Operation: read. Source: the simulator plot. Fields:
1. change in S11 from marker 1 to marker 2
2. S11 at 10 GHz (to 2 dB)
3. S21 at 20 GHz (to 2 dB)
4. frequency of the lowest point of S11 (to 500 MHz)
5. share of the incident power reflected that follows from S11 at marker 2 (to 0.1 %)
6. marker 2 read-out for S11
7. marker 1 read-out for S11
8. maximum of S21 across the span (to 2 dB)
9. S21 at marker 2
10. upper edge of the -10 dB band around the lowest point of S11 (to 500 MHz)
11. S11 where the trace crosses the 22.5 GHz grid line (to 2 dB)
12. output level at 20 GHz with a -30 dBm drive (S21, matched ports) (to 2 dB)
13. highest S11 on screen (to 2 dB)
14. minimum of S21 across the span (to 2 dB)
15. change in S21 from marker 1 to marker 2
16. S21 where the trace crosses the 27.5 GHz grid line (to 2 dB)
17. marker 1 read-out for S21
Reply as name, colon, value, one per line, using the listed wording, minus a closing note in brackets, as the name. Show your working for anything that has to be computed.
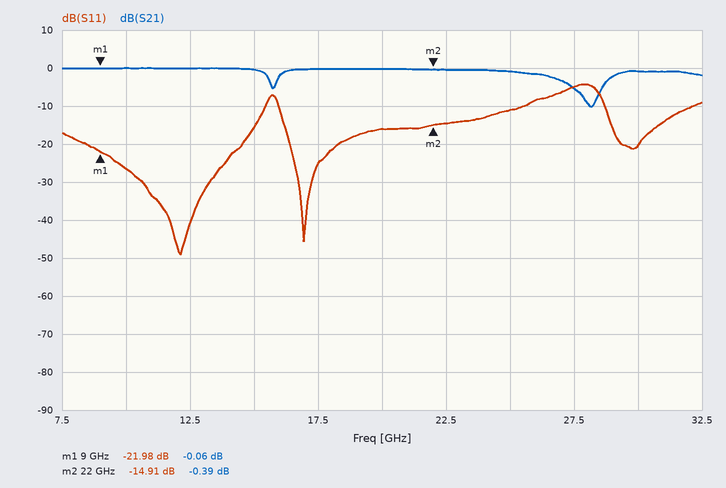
change in S11 from marker 1 to marker 2: -14.91 − (-21.98) = 7.07 dB
S11 at 10 GHz: -26 dB
S21 at 20 GHz: 0 dB
frequency of the lowest point of S11: 12.0 GHz
share of the incident power reflected that follows from S11 at marker 2: 10^(-14.91/10) ≈ 3.2 %
marker 2 read-out for S11: -14.91 dB
marker 1 read-out for S11: -21.98 dB
maximum of S21 across the span: 0 dB
S21 at marker 2: -0.39 dB
upper edge of the -10 dB band around the lowest point of S11: 15.5 GHz
S11 where the trace crosses the 22.5 GHz grid line: -14 dB
output level at 20 GHz with a -30 dBm drive (S21, matched ports): -30 dBm + (0 dB) = -30 dBm
highest S11 on screen: -4 dB
minimum of S21 across the span: -10 dB
change in S21 from marker 1 to marker 2: -0.39 − (-0.06) = -0.33 dB
S21 where the trace crosses the 27.5 GHz grid line: -6 dB
marker 1 read-out for S21: -0.06 dB
